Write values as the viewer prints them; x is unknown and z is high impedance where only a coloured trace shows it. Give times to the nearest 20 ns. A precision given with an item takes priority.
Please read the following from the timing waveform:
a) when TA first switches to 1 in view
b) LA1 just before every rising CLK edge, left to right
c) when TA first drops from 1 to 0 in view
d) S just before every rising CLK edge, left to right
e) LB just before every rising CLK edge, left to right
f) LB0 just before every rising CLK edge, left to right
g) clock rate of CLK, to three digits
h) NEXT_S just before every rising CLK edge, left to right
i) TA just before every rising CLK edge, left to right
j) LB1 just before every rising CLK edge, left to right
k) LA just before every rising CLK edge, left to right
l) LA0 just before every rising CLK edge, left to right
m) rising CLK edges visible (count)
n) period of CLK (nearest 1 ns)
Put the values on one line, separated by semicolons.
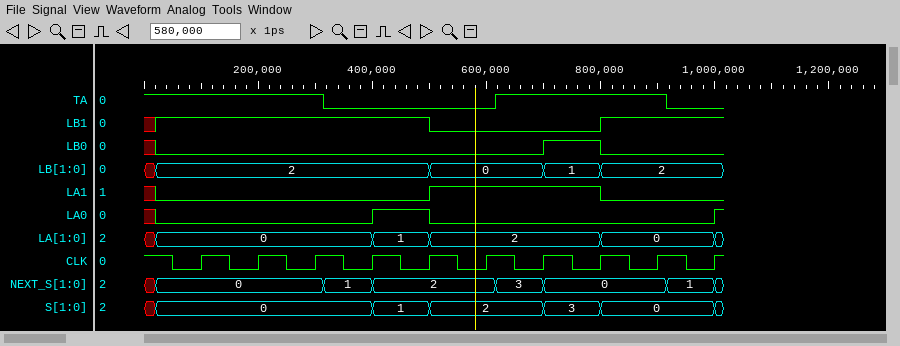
620 ns; 0 0 0 0 0 1 1 1 0 0; 320 ns; 0, 0, 0, 0, 1, 2, 2, 3, 0, 0; 2, 2, 2, 2, 2, 0, 0, 1, 2, 2; 0 0 0 0 0 0 0 1 0 0; 10.0 MHz; 0, 0, 0, 1, 2, 2, 3, 0, 0, 1; 1 1 1 0 0 0 1 1 1 0; 1 1 1 1 1 0 0 0 1 1; 0, 0, 0, 0, 1, 2, 2, 2, 0, 0; 0 0 0 0 1 0 0 0 0 0; 10; 100 ns
